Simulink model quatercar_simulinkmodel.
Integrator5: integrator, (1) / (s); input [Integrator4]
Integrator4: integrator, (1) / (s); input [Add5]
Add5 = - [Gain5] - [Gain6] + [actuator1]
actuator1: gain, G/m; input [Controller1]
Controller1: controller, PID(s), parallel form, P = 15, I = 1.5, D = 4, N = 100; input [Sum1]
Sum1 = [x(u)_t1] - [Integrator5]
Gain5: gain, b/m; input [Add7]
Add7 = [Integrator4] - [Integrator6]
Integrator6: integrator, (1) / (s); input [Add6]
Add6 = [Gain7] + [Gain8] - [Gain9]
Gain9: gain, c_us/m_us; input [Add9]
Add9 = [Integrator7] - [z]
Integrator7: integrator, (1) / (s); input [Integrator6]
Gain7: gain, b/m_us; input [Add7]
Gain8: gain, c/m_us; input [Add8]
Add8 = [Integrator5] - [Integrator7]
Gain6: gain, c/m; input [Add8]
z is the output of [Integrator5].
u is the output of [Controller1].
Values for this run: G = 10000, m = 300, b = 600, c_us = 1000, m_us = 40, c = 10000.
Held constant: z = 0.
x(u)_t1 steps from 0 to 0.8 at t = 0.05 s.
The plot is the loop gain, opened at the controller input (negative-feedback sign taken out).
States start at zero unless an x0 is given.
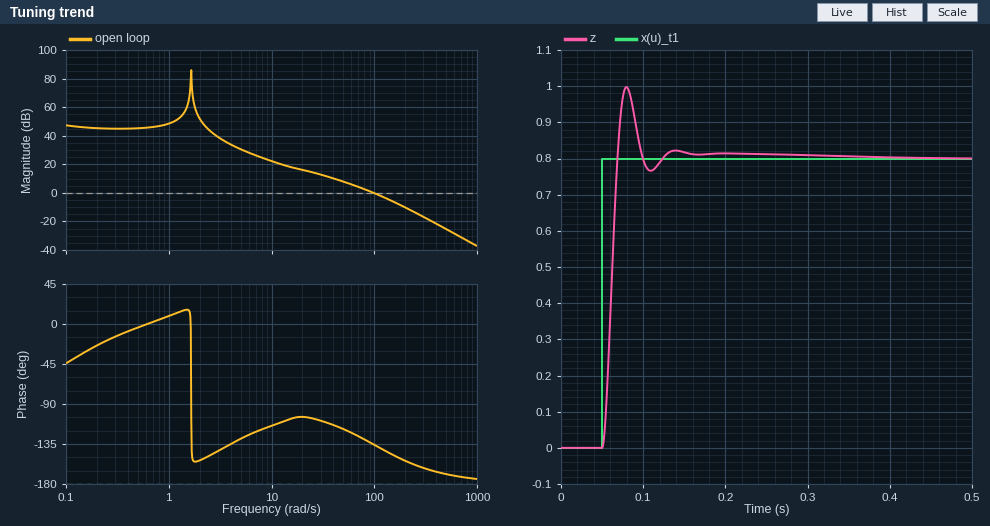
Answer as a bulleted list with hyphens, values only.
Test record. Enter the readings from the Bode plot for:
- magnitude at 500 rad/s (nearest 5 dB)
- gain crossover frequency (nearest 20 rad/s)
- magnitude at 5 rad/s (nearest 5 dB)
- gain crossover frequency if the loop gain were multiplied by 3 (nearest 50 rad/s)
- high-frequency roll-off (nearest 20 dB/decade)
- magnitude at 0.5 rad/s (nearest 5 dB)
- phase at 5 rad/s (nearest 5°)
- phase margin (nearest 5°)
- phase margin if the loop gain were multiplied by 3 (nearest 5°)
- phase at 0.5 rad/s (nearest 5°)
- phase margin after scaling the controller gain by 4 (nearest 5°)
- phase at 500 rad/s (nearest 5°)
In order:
- -25 dB
- 100 rad/s
- 30 dB
- 200 rad/s
- -40 dB/decade
- 45 dB
- -130°
- 45°
- 25°
- -5°
- 25°
- -170°
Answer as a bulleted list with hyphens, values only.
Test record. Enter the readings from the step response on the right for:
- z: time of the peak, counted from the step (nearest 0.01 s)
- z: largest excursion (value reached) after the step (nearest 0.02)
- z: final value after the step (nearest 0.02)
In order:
- 0.03 s
- 1.00
- 0.80
